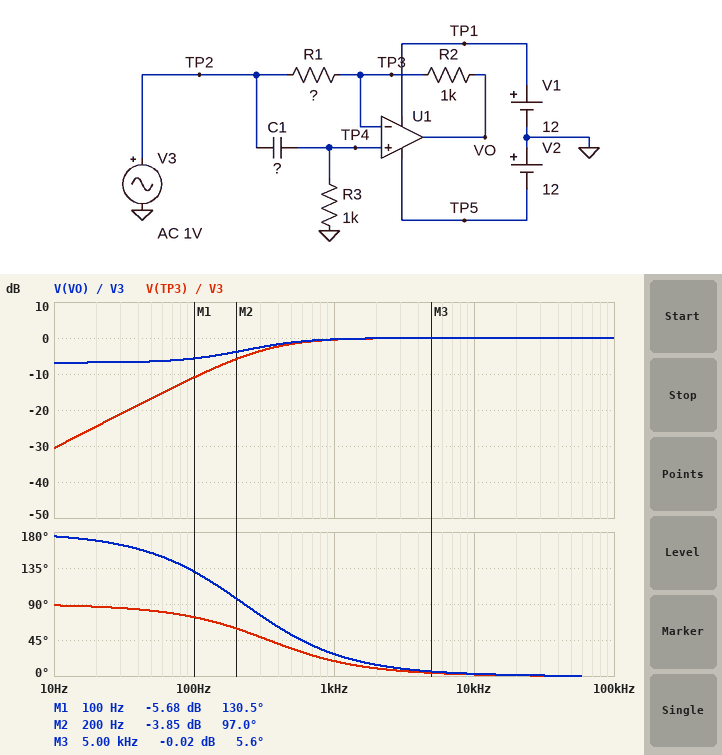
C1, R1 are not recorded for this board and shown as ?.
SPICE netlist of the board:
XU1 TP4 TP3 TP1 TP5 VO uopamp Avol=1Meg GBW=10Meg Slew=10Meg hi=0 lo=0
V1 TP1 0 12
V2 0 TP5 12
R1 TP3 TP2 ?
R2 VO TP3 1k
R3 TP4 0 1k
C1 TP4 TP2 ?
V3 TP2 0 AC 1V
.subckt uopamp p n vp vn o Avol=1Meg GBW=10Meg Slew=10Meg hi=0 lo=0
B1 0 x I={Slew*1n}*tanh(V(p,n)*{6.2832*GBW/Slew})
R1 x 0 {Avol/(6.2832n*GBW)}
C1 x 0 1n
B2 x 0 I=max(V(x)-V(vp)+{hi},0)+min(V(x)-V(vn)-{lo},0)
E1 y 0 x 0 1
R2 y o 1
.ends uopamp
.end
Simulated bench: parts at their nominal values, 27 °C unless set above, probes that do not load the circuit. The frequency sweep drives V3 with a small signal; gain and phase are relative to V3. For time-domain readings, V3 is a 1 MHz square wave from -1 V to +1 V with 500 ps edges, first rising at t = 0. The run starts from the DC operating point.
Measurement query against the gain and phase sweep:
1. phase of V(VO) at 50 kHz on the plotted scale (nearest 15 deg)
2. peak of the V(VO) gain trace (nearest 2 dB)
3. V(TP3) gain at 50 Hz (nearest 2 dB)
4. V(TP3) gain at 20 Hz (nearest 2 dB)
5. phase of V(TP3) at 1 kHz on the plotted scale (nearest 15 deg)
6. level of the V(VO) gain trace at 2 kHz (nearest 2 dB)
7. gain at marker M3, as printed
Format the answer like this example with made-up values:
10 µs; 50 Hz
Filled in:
0 deg; 0 dB; -16 dB; -24 dB; 15 deg; 0 dB; -0.02 dB
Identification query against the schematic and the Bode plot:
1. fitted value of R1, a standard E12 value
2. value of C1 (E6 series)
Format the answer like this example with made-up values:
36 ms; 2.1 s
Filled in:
2.2 kΩ; 470 nF
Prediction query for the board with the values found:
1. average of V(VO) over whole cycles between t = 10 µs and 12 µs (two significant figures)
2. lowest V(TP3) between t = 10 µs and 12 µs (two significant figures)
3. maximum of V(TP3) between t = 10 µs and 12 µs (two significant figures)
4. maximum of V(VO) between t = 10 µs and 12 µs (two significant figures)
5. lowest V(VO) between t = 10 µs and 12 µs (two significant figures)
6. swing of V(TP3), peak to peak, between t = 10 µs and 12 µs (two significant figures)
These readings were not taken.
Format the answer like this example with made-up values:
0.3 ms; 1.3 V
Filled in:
1.4 V; -25 mV; 2.0 V; 2.4 V; 420 mV; 2.0 V
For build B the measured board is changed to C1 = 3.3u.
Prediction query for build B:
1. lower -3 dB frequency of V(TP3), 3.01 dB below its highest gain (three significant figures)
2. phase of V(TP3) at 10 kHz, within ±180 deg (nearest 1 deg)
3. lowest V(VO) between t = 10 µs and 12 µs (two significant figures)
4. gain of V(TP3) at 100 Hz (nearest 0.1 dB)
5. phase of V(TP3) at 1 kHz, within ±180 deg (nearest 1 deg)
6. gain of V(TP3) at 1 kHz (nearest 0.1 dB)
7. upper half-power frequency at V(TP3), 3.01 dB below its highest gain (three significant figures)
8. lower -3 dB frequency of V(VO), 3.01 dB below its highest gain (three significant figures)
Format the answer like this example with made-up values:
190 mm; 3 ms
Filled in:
48.2 Hz; 0 deg; 450 mV; -0.9 dB; 3 deg; 0 dB; 7.66 MHz; 36.9 Hz
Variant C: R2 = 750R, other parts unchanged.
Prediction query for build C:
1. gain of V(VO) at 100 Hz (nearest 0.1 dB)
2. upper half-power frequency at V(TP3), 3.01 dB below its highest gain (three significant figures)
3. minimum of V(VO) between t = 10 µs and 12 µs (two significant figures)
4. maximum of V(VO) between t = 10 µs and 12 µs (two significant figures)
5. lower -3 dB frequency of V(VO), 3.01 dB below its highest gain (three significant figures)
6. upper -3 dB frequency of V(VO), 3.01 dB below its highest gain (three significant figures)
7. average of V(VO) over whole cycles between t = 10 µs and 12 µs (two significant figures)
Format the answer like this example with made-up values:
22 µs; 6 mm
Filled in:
-7.3 dB; 7.99 MHz; 310 mV; 2.3 V; 297 Hz; 7.46 MHz; 1.3 V
